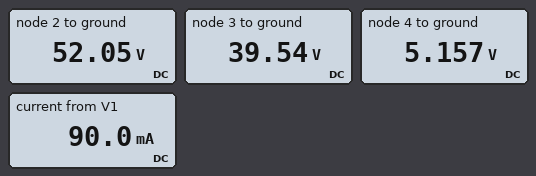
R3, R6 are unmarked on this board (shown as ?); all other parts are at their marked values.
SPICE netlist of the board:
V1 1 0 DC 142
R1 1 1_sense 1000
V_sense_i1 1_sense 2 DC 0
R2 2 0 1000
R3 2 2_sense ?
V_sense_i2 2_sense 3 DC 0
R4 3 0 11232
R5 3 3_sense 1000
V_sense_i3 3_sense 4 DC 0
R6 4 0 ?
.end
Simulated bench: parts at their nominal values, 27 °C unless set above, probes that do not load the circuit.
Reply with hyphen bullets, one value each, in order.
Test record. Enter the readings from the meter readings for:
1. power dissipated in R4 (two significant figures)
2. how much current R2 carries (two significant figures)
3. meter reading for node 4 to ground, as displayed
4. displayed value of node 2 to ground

- 140 mW
- 52 mA
- 5.157 V
- 52.05 V
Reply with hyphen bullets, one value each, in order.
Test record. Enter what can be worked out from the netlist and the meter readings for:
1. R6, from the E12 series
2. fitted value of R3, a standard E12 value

- 150 Ω
- 330 Ω
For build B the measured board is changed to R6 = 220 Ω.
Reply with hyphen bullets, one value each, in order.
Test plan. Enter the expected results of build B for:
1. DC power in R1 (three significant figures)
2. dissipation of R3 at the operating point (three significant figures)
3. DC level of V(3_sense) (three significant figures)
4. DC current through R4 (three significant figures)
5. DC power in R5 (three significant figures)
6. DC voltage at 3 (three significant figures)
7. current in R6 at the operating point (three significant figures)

- 7.99 W
- 446 mW
- 7.30 V
- 3.60 mA
- 1.10 W
- 40.5 V
- 33.2 mA
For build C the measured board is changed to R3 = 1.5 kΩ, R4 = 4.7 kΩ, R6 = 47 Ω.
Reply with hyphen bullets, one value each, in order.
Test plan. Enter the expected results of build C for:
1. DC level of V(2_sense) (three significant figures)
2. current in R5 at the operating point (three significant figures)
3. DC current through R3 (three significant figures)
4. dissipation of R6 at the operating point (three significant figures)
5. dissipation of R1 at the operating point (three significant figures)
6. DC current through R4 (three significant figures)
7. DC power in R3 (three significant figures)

- 21.3 V
- 20.3 mA
- 24.9 mA
- 19.4 mW
- 6.96 W
- 4.53 mA
- 927 mW
